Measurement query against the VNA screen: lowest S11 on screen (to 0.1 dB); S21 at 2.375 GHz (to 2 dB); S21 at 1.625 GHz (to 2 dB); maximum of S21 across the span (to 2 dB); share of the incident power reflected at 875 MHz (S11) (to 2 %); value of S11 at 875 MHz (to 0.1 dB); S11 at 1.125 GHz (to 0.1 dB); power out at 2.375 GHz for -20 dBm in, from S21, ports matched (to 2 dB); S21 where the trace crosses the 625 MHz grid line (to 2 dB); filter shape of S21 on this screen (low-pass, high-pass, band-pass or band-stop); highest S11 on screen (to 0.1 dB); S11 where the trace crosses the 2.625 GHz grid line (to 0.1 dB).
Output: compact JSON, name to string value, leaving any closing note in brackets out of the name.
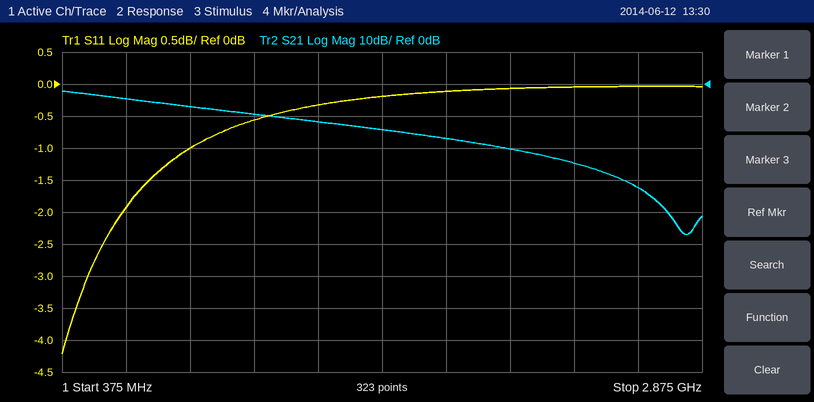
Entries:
{"lowest S11 on screen": "-4.2 dB", "S21 at 2.375 GHz": "-24 dB", "S21 at 1.625 GHz": "-14 dB", "maximum of S21 across the span": "-2 dB", "share of the incident power reflected at 875 MHz (S11)": "80 %", "value of S11 at 875 MHz": "-1.0 dB", "S11 at 1.125 GHz": "-0.6 dB", "power out at 2.375 GHz for -20 dBm in, from S21, ports matched": "-44 dBm", "S21 where the trace crosses the 625 MHz grid line": "-4 dB", "filter shape of S21 on this screen": "low-pass", "highest S11 on screen": "0.0 dB", "S11 where the trace crosses the 2.625 GHz grid line": "0.0 dB"}
